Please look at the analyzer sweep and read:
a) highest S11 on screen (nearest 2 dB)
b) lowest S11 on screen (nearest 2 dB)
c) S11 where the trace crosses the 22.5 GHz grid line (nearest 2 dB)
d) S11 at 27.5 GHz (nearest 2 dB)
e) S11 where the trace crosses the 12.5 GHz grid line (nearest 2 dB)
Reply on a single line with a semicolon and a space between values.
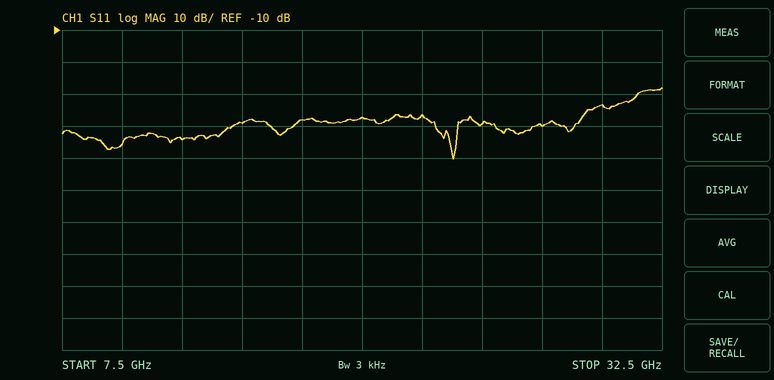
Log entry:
-28 dB; -50 dB; -36 dB; -40 dB; -44 dB
